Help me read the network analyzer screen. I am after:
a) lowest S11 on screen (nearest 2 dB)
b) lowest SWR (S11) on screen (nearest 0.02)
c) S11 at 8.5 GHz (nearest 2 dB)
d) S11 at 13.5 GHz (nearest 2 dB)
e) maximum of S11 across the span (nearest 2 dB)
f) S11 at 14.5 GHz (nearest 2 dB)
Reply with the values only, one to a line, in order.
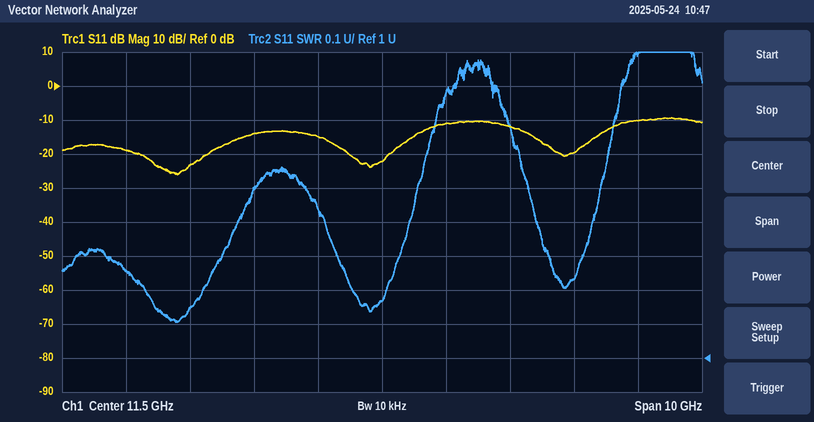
-26 dB
1.10
-24 dB
-12 dB
-10 dB
-20 dB
